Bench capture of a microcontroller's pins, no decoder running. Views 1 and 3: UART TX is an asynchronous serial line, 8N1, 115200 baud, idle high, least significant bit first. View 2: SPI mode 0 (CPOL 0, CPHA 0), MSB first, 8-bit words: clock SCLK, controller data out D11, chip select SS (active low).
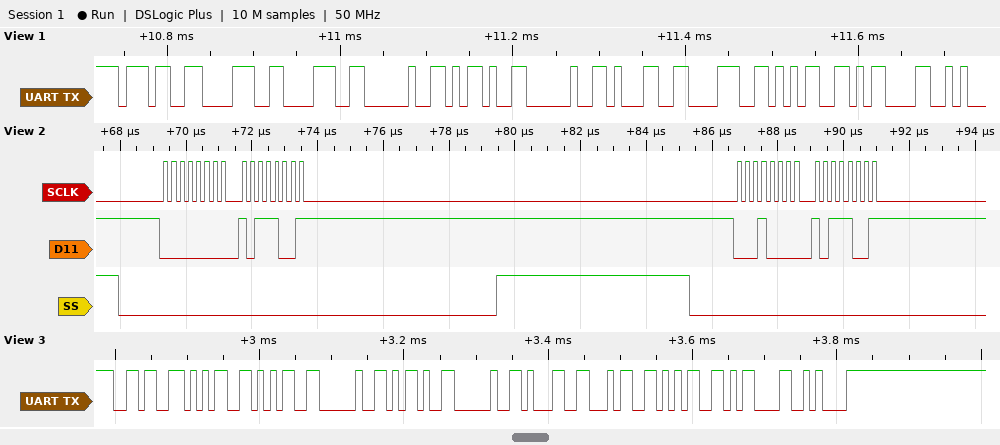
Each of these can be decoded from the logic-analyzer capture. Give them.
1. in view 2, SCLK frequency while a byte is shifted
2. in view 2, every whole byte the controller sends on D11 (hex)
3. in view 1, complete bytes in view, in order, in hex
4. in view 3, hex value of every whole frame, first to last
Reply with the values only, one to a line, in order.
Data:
4 MHz
00 B9 10 B9
37 38 38 20 2D 20 31 38 35 0D
36 35 35 20 2D 20 31 34 35 0D 0A
